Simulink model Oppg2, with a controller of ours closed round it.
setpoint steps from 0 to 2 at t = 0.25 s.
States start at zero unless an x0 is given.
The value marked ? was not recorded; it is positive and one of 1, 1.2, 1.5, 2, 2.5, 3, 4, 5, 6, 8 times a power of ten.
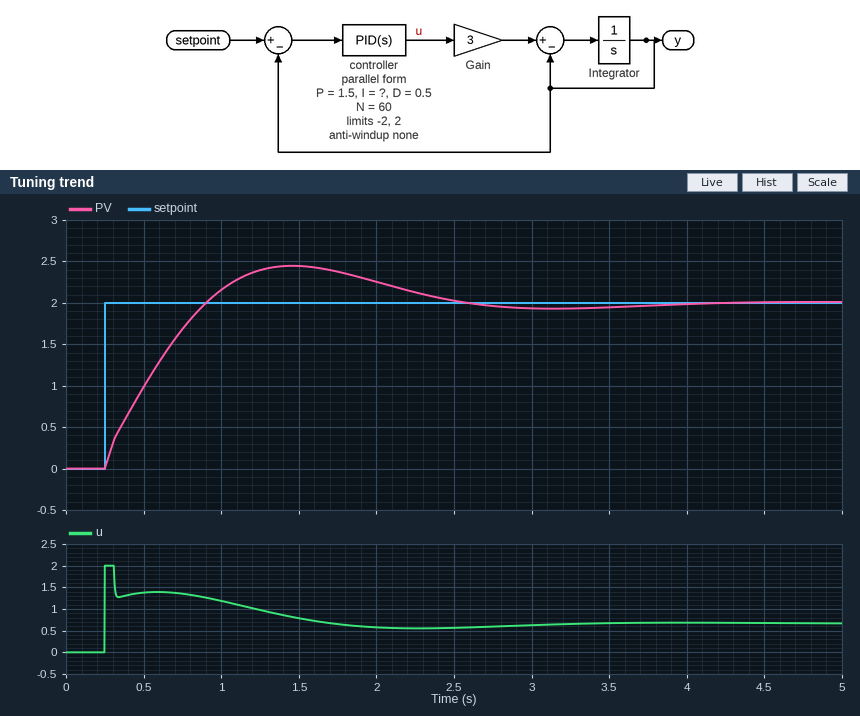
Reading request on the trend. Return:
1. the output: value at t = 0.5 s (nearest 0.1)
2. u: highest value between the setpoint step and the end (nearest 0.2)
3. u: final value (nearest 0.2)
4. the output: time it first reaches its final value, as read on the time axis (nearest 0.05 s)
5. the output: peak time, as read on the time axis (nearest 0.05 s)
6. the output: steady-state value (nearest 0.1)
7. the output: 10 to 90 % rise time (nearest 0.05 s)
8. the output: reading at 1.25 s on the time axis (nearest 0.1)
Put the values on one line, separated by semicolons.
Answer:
1.0; 2.0; 0.6; 0.90 s; 1.45 s; 2.0; 0.50 s; 2.4
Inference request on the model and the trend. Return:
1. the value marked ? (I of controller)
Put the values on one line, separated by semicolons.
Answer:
4
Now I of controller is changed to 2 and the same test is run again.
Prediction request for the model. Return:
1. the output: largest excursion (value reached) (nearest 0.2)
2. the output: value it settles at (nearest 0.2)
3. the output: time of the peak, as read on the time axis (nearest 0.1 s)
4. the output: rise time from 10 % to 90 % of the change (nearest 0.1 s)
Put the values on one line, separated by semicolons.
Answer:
2.2; 2.0; 1.9 s; 0.7 s
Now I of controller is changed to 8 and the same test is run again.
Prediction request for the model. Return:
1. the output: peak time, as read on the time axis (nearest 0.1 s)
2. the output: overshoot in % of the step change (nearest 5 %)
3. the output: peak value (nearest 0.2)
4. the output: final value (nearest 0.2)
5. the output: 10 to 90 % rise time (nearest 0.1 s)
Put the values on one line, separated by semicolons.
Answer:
1.1 s; 35 %; 2.6; 2.0; 0.4 s
